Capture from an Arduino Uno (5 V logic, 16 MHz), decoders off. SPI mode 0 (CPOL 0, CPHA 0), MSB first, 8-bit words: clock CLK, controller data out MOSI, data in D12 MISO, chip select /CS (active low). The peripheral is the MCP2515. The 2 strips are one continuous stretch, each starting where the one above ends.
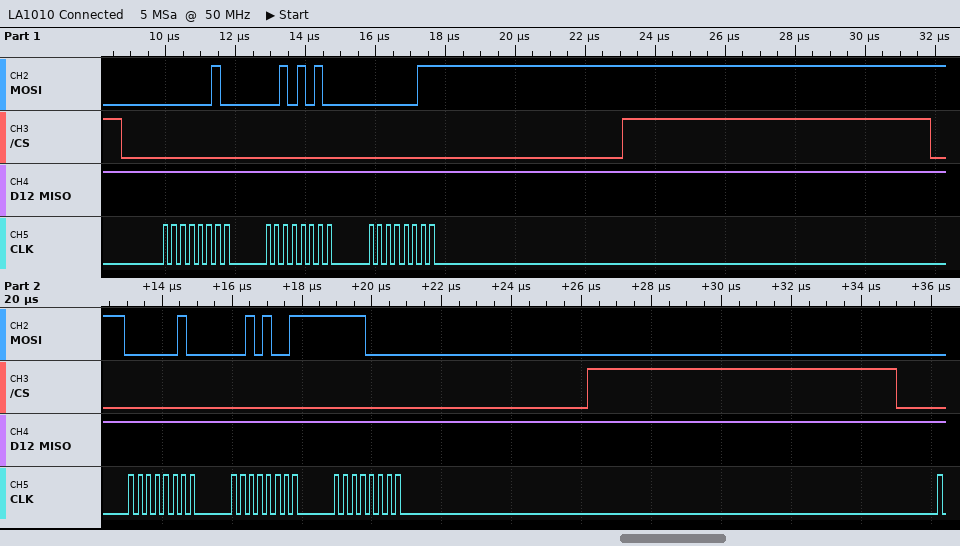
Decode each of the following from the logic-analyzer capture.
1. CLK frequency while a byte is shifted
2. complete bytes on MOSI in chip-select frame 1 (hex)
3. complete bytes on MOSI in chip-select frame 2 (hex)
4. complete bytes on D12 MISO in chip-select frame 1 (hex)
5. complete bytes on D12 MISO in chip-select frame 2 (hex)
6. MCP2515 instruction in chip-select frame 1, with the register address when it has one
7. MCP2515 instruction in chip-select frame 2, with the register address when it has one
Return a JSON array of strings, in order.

["4 MHz", "02 2A 03", "02 29 F0", "FF FF FF", "FF FF FF", "WRITE 0x2A", "WRITE 0x29"]
